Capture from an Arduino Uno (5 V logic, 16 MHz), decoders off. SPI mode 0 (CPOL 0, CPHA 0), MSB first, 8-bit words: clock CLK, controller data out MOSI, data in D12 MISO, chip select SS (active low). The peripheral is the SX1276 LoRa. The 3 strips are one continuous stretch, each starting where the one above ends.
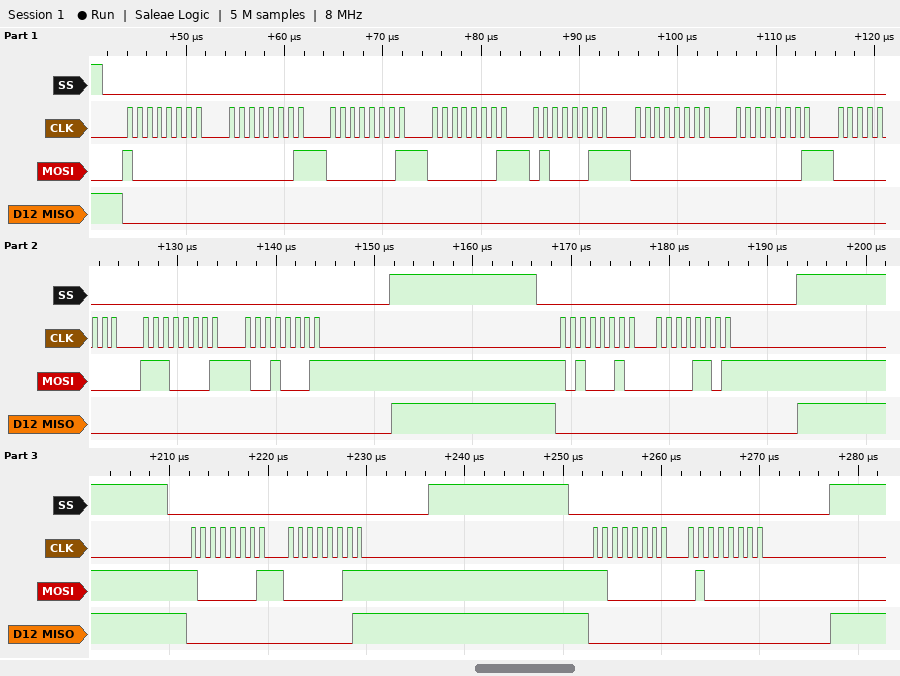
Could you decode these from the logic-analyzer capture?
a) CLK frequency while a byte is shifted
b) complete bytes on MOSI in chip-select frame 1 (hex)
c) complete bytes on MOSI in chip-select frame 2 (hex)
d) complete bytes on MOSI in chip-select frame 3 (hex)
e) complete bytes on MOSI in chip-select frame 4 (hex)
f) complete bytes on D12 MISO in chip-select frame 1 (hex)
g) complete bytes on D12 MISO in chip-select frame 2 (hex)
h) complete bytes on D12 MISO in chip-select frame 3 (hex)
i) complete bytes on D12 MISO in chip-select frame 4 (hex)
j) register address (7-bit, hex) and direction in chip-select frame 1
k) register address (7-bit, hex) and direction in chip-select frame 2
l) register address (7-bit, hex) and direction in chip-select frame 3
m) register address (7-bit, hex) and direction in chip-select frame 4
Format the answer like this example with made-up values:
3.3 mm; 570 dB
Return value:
1 MHz; 80 01 01 01 43 00 01 00 E1 91; A2 0D; 81 03; C0 40; 00 00 00 00 00 00 00 00 00 00; 00 00; 00 01; 00 00; 0x00 write; 0x22 write; 0x01 write; 0x40 write
